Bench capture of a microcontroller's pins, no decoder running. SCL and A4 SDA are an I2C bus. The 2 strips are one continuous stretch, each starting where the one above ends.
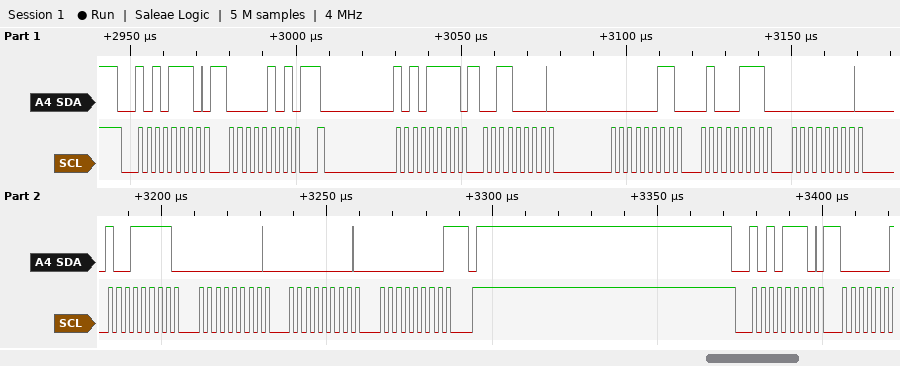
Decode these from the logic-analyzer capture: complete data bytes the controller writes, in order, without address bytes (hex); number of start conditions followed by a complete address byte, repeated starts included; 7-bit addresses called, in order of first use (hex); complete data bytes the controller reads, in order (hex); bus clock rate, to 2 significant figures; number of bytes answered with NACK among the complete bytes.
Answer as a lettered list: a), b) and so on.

a) 05
b) 3
c) 0x57
d) 30 03 47 00 9F 00 00 00
e) 400 kHz
f) 1
